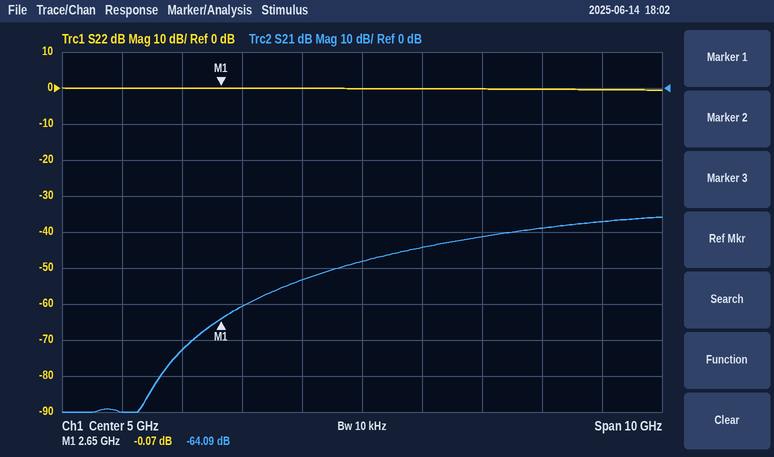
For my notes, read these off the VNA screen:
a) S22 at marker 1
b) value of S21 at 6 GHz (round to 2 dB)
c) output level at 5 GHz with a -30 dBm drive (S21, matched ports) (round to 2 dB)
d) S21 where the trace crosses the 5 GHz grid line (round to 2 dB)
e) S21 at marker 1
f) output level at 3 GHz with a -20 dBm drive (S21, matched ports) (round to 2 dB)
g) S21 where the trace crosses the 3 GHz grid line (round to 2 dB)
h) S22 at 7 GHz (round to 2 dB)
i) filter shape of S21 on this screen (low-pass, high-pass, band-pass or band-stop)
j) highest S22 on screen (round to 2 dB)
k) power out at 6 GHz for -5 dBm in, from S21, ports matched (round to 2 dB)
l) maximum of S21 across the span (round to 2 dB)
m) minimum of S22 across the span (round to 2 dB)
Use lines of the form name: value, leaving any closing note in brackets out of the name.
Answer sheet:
S22 at marker 1: -0.07 dB
value of S21 at 6 GHz: -44 dB
output level at 5 GHz with a -30 dBm drive (S21, matched ports): -78 dBm
S21 where the trace crosses the 5 GHz grid line: -48 dB
S21 at marker 1: -64.09 dB
output level at 3 GHz with a -20 dBm drive (S21, matched ports): -80 dBm
S21 where the trace crosses the 3 GHz grid line: -60 dB
S22 at 7 GHz: 0 dB
filter shape of S21 on this screen: high-pass
highest S22 on screen: 0 dB
power out at 6 GHz for -5 dBm in, from S21, ports matched: -50 dBm
maximum of S21 across the span: -36 dB
minimum of S22 across the span: 0 dB
